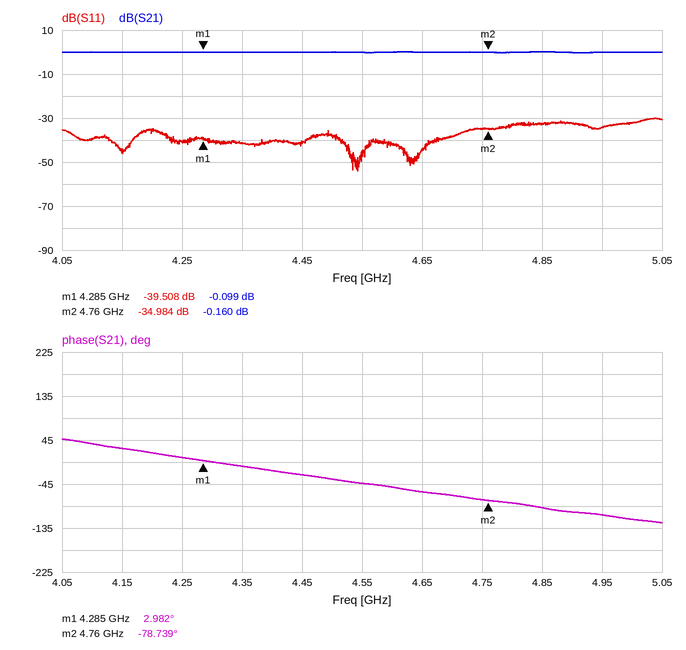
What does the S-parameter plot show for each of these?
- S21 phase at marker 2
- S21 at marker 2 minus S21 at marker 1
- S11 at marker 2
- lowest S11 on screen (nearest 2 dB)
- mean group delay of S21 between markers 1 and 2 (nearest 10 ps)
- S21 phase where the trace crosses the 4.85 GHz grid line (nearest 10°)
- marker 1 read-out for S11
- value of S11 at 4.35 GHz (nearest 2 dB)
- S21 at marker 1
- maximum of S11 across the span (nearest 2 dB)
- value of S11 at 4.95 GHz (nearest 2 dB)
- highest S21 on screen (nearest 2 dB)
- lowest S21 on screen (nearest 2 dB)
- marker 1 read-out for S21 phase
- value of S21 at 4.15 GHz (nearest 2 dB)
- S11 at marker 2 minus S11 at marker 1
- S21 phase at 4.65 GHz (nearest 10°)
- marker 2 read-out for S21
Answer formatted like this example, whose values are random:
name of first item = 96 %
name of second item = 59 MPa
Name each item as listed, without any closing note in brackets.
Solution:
S21 phase at marker 2 = -78.739°
S21 at marker 2 minus S21 at marker 1 = -0.061 dB
S11 at marker 2 = -34.984 dB
lowest S11 on screen = -54 dB
mean group delay of S21 between markers 1 and 2 = 480 ps
S21 phase where the trace crosses the 4.85 GHz grid line = -90°
marker 1 read-out for S11 = -39.508 dB
value of S11 at 4.35 GHz = -42 dB
S21 at marker 1 = -0.099 dB
maximum of S11 across the span = -30 dB
value of S11 at 4.95 GHz = -34 dB
highest S21 on screen = 0 dB
lowest S21 on screen = 0 dB
marker 1 read-out for S21 phase = 2.982°
value of S21 at 4.15 GHz = 0 dB
S11 at marker 2 minus S11 at marker 1 = 4.524 dB
S21 phase at 4.65 GHz = -60°
marker 2 read-out for S21 = -0.160 dB
